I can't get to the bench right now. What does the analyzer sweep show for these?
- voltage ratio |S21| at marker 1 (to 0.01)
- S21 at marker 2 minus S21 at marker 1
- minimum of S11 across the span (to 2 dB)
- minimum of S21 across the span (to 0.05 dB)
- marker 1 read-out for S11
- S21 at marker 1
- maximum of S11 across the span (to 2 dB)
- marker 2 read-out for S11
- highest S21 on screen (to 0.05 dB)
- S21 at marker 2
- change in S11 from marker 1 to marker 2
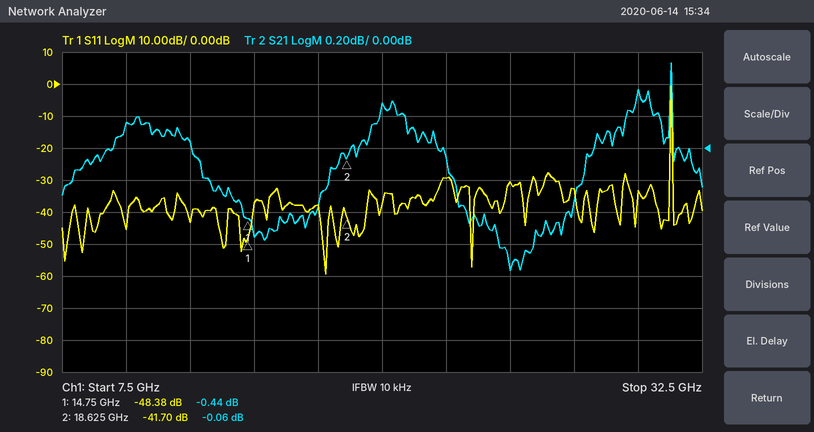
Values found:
0.95
0.38 dB
-60 dB
-0.75 dB
-48.38 dB
-0.44 dB
0 dB
-41.70 dB
0.55 dB
-0.06 dB
6.68 dB
